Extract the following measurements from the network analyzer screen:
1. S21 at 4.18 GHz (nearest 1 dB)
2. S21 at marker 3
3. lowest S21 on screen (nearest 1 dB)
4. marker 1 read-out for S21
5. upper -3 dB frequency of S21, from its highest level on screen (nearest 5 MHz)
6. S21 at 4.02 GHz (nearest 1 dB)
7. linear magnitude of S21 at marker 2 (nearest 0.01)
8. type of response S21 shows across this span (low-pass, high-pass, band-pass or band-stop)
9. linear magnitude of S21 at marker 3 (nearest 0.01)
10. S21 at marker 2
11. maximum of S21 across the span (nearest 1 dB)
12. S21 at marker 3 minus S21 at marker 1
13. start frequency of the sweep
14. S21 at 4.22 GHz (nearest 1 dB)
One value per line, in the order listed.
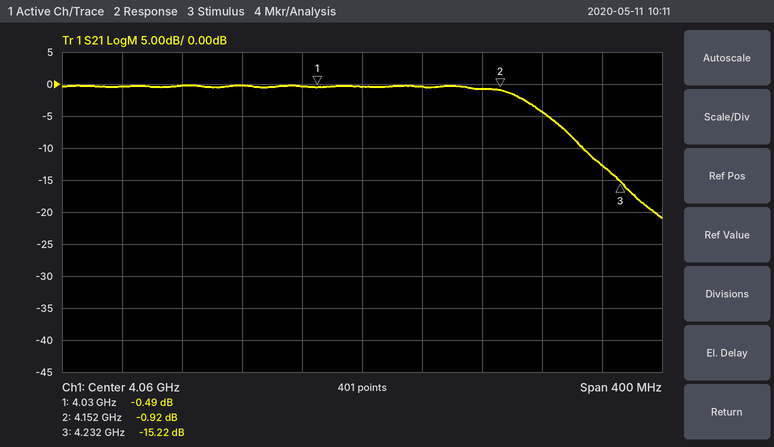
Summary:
-4 dB
-15.22 dB
-21 dB
-0.49 dB
4.175 GHz
0 dB
0.90
low-pass
0.17
-0.92 dB
0 dB
-14.73 dB
3.86 GHz
-13 dB
